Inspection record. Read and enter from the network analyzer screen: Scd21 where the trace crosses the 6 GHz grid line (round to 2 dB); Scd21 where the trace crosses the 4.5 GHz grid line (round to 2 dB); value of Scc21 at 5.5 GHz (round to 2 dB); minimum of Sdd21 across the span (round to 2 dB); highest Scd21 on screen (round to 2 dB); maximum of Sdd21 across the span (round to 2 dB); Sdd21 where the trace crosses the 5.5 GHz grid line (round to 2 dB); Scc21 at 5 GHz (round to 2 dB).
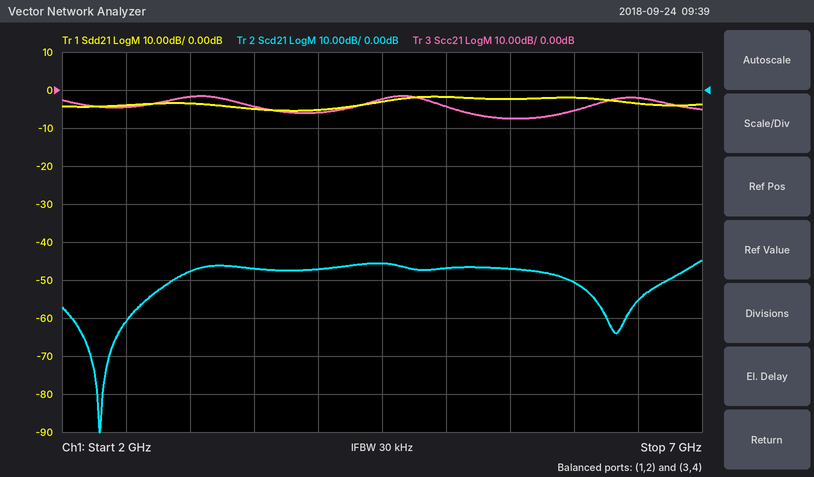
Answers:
-50 dB
-46 dB
-8 dB
-6 dB
-44 dB
-2 dB
-2 dB
-4 dB
